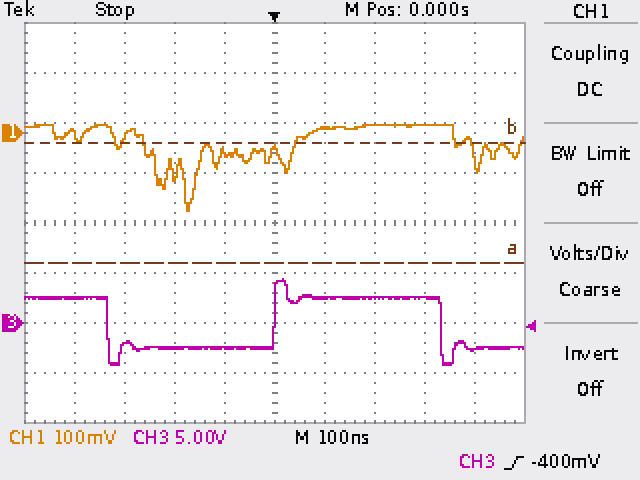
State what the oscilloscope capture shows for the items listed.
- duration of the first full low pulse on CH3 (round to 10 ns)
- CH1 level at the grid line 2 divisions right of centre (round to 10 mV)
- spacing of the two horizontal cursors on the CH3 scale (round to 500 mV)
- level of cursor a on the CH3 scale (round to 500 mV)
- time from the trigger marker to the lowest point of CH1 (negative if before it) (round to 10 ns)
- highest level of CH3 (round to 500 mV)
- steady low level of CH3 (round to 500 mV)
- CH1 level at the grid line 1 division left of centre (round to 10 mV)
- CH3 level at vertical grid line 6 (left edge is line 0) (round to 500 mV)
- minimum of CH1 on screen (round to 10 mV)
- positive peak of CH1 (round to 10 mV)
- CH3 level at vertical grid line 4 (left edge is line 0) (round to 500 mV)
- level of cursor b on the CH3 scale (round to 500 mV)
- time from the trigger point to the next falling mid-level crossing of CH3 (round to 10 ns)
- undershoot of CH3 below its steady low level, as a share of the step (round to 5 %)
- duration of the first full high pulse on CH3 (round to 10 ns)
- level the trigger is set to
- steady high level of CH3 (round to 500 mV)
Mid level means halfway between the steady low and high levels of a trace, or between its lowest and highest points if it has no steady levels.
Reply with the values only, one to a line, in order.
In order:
330 ns
20 mV
12.0 V
6.0 V
-170 ns
4.5 V
-2.5 V
-40 mV
2.5 V
-160 mV
20 mV
-2.5 V
18.0 V
330 ns
35 %
330 ns
-400 mV
2.5 V
